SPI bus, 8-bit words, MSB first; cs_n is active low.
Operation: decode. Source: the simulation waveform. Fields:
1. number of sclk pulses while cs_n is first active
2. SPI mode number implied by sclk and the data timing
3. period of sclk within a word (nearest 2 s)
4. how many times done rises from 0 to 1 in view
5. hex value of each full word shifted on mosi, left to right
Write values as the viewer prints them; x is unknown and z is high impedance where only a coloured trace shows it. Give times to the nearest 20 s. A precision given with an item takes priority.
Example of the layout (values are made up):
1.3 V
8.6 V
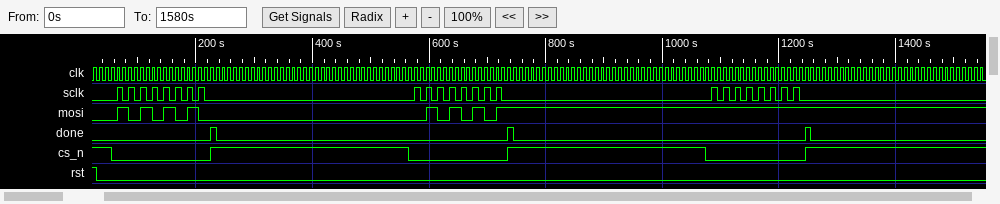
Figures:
8
1
20 s
3
AA, 55, FF
